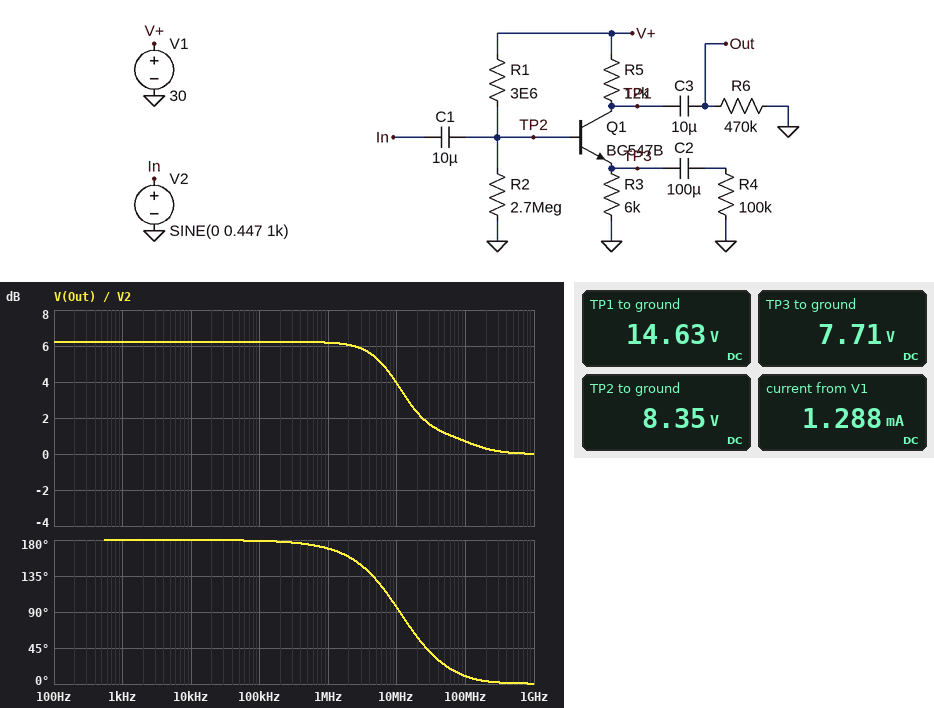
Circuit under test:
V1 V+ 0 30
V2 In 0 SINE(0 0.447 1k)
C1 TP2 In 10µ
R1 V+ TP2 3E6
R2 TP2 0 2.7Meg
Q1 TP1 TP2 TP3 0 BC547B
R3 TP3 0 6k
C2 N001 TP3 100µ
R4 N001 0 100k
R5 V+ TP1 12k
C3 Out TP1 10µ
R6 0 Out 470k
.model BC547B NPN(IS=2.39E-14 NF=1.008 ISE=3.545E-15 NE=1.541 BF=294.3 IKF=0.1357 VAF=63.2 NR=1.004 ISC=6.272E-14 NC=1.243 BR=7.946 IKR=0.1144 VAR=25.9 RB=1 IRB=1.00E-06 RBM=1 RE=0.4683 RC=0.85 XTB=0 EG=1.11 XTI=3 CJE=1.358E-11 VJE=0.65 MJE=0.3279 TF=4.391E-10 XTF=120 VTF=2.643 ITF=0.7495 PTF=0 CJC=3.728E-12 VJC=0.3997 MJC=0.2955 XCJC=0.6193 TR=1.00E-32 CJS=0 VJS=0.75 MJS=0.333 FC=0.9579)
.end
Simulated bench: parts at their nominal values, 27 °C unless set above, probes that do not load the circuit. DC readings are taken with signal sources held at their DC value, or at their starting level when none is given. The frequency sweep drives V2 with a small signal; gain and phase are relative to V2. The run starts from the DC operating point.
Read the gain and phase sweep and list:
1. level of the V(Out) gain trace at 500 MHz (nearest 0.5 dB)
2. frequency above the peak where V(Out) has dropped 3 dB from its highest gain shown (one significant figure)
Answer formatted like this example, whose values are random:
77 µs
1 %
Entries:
0 dB
10 MHz
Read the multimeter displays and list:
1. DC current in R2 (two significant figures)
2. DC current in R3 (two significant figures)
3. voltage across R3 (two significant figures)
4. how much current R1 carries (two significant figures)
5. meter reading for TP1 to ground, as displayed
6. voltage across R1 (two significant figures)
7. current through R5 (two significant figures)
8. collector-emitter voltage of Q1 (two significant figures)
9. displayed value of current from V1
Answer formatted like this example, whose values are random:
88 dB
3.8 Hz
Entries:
3.1 µA
1.3 mA
7.7 V
7.2 µA
14.63 V
22 V
1.3 mA
6.9 V
1.288 mA
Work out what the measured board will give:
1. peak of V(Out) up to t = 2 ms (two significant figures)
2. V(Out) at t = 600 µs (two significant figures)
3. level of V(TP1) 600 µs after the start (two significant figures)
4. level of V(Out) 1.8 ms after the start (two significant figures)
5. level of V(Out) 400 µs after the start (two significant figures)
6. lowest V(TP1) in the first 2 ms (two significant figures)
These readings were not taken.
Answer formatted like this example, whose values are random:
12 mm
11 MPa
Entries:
920 mV
540 mV
15 V
870 mV
-540 mV
14 V
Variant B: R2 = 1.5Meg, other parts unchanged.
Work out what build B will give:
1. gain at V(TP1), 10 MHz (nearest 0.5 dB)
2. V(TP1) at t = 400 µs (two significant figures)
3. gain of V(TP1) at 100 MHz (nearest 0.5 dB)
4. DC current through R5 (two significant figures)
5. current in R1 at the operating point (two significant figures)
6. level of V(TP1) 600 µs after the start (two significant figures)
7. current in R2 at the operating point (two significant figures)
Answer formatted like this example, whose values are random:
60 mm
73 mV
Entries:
4.5 dB
17 V
1.0 dB
1.0 mA
7.7 µA
18 V
4.6 µA
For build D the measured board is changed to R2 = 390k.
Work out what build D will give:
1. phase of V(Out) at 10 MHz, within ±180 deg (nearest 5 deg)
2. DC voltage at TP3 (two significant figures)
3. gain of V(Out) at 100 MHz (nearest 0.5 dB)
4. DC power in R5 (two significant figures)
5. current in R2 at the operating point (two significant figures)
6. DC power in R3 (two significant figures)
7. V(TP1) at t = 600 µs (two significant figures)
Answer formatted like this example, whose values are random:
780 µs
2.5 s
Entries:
110 deg
2.5 V
1.0 dB
2.0 mW
7.9 µA
1.0 mW
26 V
